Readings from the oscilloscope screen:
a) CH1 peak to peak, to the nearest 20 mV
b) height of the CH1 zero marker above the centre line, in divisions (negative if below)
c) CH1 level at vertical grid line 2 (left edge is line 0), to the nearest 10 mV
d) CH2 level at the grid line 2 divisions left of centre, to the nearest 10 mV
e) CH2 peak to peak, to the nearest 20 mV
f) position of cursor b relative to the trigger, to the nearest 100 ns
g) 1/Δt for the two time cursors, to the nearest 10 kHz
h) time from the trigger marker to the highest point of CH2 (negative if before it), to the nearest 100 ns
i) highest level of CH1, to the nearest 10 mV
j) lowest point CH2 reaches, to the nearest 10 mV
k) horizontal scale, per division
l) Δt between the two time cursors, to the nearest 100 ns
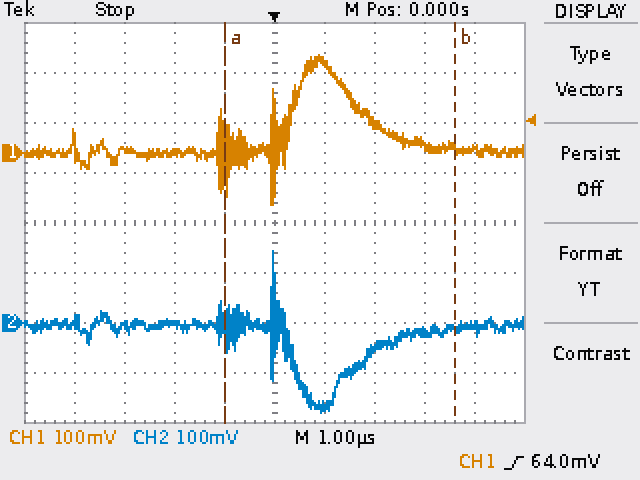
300 mV
+1.4 div
10 mV
0 mV
320 mV
+3.6 µs
220 kHz
0.0 µs
200 mV
-180 mV
1 µs
4.6 µs
